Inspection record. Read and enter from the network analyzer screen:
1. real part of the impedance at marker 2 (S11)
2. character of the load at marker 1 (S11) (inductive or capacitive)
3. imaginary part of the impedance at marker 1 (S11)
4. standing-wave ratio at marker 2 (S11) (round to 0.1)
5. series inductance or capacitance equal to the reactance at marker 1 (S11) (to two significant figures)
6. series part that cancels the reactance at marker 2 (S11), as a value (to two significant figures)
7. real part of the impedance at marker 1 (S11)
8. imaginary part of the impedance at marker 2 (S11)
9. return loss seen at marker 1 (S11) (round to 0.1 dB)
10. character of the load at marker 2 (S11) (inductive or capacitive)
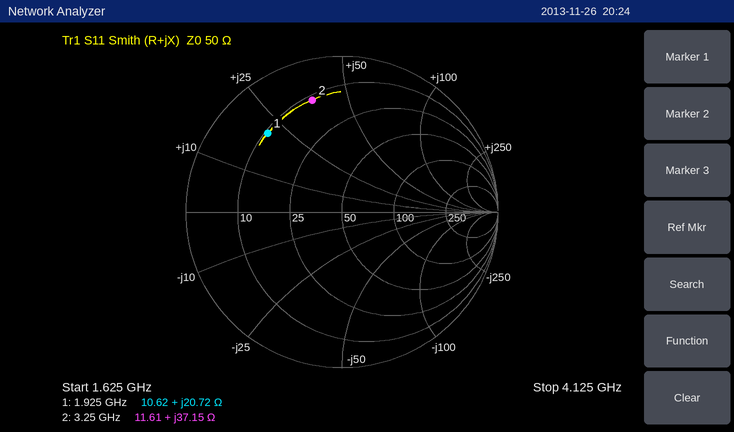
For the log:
11.61 Ω
inductive
+20.72 Ω
6.8
1.7 nH
1.3 pF
10.62 Ω
+37.15 Ω
3.2 dB
inductive
